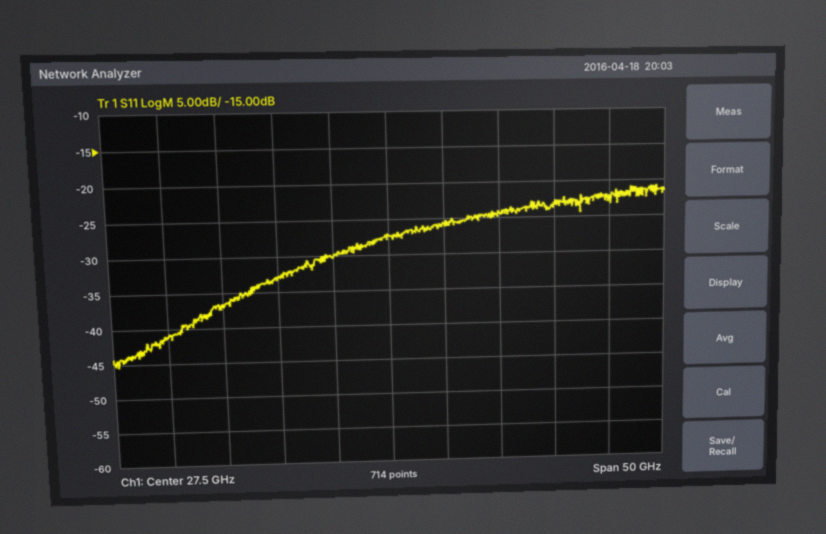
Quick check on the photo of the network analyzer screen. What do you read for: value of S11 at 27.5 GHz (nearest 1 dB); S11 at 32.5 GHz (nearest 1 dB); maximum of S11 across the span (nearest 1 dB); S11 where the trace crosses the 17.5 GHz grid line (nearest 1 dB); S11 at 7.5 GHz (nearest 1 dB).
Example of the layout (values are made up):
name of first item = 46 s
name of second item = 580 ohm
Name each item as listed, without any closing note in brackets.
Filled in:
value of S11 at 27.5 GHz = -27 dB
S11 at 32.5 GHz = -26 dB
maximum of S11 across the span = -21 dB
S11 where the trace crosses the 17.5 GHz grid line = -33 dB
S11 at 7.5 GHz = -41 dB
